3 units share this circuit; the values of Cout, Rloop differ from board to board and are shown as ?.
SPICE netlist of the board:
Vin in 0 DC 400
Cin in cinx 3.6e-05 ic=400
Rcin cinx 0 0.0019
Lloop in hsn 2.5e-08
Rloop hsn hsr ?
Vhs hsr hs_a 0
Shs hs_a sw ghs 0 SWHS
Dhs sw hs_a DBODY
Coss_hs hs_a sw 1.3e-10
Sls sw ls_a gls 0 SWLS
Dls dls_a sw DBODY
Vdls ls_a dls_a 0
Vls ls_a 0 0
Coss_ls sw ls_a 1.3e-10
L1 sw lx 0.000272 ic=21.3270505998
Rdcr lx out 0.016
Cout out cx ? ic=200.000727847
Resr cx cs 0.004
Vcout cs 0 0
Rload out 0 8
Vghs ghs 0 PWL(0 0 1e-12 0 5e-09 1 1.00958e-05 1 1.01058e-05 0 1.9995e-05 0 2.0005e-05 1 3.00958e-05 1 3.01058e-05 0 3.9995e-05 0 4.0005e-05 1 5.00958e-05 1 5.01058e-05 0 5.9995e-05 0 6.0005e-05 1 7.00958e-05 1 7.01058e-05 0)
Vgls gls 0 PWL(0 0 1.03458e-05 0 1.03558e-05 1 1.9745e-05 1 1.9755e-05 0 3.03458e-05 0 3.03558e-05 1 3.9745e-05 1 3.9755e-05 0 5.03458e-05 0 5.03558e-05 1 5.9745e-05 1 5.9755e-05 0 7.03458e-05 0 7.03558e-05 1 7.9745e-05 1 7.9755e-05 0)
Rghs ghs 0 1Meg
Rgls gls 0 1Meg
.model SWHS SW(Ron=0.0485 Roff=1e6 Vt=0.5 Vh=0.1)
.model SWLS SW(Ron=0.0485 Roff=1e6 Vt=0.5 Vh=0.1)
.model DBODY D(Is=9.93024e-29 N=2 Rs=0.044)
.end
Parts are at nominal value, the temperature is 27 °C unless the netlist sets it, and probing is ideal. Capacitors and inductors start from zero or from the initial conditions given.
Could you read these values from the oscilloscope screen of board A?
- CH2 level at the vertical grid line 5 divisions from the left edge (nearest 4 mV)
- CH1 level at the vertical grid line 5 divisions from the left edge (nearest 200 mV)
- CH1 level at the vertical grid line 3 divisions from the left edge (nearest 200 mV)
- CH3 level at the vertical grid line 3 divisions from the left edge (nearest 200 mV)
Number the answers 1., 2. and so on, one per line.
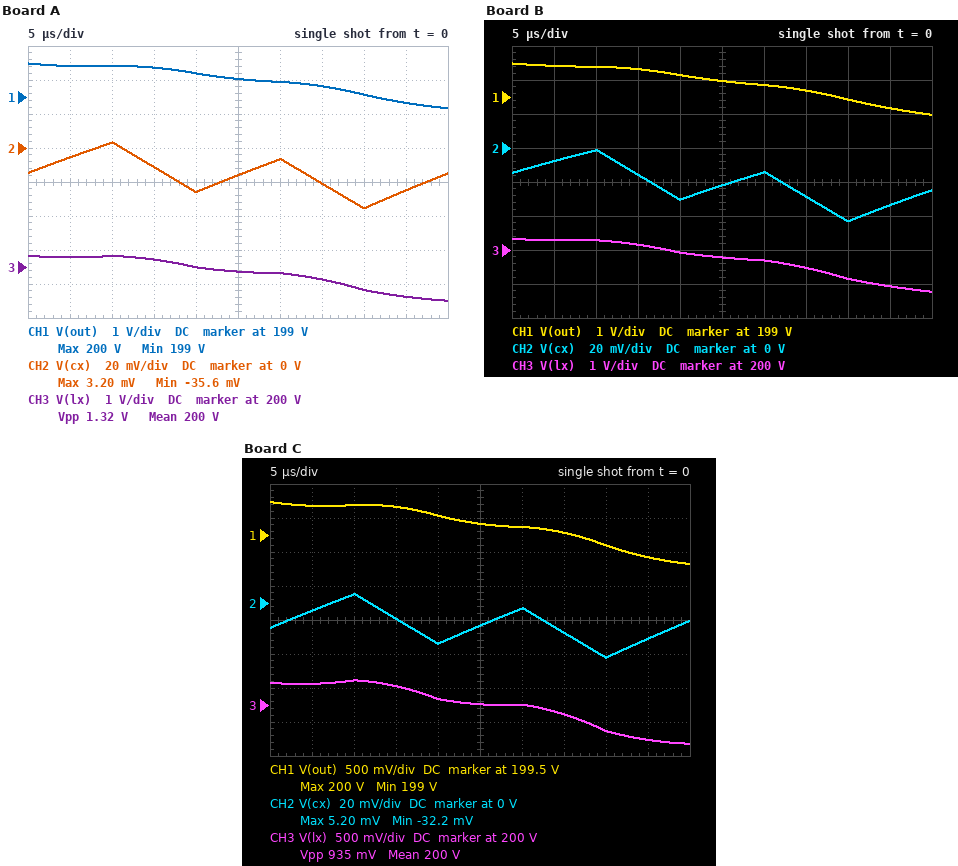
1. -16 mV
2. 199.6 V
3. 199.8 V
4. 200.2 V
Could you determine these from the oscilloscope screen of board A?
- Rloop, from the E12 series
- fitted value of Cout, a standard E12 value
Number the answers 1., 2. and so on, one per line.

1. 3.3 Ω
2. 150 µF
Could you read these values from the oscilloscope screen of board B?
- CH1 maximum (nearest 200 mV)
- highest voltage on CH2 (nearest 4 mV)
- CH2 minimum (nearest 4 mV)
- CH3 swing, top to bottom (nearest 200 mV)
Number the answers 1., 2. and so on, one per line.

1. 200.0 V
2. 0 V
3. -44 mV
4. 1.6 V
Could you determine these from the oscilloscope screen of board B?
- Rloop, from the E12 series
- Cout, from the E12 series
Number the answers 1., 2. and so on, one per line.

1. 4.7 Ω
2. 180 µF
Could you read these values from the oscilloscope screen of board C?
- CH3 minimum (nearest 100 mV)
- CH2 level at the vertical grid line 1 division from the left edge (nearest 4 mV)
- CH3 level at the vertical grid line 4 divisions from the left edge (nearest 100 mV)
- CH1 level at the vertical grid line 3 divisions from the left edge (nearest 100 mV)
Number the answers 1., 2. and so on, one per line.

1. 199.4 V
2. -4 mV
3. 200.1 V
4. 199.9 V
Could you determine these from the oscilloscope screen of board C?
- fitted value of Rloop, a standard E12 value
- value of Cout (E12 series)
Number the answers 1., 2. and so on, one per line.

1. 2.7 Ω
2. 180 µF
